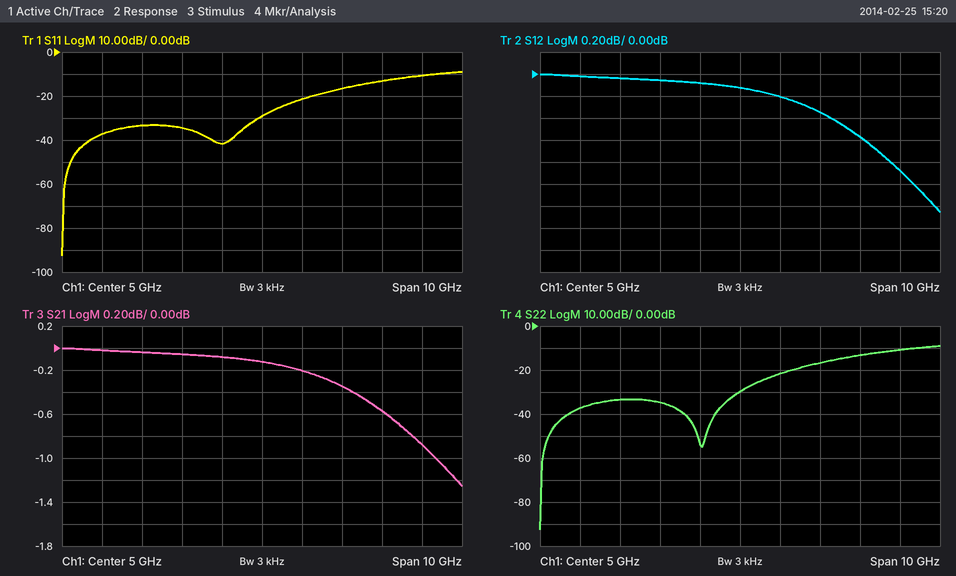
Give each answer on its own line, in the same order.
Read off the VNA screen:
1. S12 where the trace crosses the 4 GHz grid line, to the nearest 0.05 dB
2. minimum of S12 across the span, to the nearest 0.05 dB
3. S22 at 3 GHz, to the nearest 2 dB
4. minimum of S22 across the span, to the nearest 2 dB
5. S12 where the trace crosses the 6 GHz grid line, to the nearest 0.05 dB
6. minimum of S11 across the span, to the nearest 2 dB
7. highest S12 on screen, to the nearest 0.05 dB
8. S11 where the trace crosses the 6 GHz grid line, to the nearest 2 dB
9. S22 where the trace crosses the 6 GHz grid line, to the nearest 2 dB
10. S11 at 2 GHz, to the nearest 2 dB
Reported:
-0.10 dB
-1.25 dB
-34 dB
-92 dB
-0.20 dB
-92 dB
0.00 dB
-22 dB
-22 dB
-34 dB
